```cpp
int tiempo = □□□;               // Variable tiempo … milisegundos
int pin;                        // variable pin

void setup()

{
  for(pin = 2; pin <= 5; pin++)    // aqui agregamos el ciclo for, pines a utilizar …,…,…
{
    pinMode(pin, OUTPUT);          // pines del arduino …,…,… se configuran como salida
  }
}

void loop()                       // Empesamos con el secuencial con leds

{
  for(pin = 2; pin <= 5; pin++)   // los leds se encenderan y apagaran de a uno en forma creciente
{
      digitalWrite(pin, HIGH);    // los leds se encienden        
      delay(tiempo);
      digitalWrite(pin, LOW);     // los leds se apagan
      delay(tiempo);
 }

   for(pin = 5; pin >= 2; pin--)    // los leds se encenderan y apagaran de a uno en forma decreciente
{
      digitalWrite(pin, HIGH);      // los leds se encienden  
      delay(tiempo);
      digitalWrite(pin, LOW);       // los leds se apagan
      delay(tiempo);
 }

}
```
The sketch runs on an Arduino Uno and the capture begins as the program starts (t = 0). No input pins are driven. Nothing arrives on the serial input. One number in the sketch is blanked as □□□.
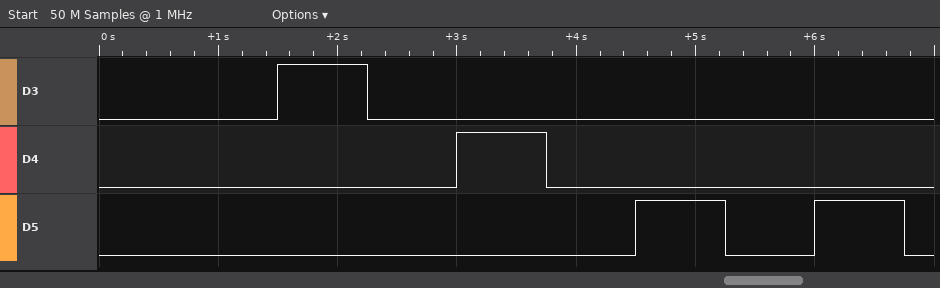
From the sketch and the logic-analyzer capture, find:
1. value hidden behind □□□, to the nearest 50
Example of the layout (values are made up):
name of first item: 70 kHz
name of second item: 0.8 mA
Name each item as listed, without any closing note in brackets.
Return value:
value hidden behind □□□, to the nearest 50: 750
